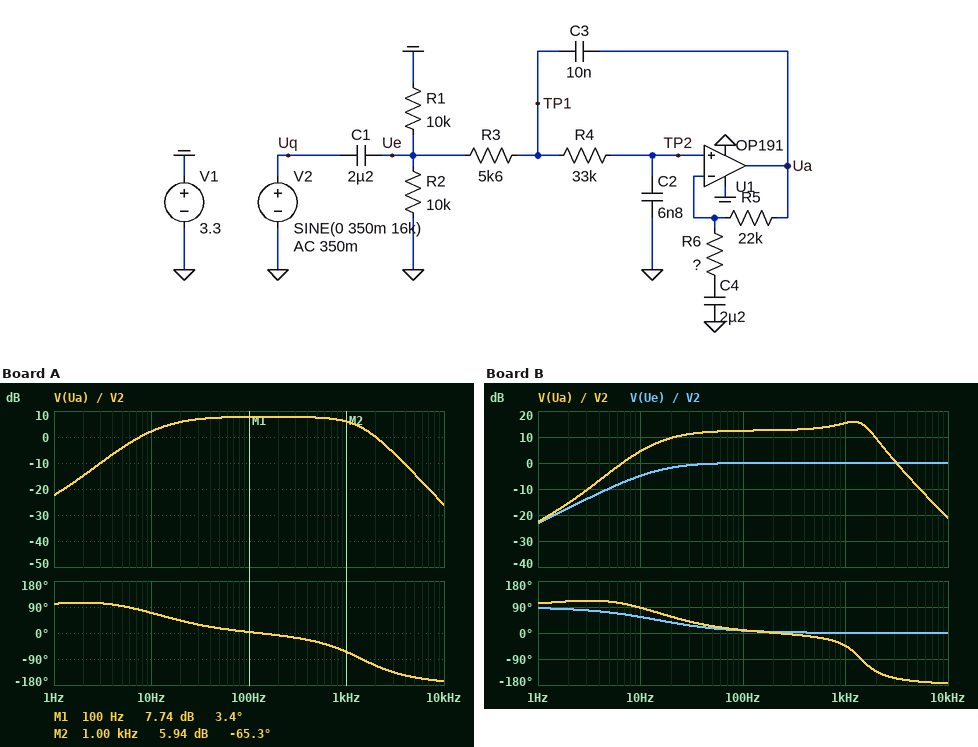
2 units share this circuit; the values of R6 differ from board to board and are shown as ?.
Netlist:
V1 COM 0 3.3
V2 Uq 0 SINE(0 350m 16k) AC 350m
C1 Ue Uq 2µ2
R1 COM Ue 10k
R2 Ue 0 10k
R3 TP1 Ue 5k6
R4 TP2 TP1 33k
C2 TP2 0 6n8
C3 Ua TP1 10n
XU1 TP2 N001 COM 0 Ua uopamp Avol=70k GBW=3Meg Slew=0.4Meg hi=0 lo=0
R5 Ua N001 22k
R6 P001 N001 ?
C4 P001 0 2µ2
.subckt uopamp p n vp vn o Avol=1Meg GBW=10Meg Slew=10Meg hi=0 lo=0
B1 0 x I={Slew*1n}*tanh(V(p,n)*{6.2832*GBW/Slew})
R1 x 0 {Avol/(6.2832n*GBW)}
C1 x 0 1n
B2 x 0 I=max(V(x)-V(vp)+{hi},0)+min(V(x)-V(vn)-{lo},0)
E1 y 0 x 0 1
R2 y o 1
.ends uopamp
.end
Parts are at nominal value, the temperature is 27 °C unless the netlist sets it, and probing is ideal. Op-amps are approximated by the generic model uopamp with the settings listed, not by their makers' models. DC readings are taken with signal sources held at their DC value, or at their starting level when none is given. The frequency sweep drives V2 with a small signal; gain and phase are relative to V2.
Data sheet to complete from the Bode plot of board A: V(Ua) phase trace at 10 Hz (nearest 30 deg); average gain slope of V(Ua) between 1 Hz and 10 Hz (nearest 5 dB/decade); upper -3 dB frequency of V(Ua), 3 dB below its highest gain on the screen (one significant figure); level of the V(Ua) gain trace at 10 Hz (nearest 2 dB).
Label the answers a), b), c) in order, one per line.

a) 60 deg
b) 25 dB/decade
c) 1 kHz
d) 2 dB
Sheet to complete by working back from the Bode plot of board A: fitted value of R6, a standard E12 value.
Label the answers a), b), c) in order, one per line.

a) 15 kΩ
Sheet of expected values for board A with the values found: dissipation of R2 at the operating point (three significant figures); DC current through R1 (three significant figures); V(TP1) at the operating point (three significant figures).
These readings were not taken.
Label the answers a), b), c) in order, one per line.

a) 272 µW
b) 165 µA
c) 1.65 V
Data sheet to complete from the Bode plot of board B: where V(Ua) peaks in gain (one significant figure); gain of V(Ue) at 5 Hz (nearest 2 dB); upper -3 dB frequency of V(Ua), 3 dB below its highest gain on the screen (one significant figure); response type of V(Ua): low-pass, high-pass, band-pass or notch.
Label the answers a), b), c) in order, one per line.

a) 1 kHz
b) -10 dB
c) 2 kHz
d) band-pass
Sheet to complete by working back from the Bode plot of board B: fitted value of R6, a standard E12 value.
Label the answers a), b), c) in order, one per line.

a) 6.8 kΩ
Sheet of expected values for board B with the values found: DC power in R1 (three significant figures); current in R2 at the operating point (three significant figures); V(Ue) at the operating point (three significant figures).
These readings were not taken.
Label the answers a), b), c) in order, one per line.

a) 272 µW
b) 165 µA
c) 1.65 V
